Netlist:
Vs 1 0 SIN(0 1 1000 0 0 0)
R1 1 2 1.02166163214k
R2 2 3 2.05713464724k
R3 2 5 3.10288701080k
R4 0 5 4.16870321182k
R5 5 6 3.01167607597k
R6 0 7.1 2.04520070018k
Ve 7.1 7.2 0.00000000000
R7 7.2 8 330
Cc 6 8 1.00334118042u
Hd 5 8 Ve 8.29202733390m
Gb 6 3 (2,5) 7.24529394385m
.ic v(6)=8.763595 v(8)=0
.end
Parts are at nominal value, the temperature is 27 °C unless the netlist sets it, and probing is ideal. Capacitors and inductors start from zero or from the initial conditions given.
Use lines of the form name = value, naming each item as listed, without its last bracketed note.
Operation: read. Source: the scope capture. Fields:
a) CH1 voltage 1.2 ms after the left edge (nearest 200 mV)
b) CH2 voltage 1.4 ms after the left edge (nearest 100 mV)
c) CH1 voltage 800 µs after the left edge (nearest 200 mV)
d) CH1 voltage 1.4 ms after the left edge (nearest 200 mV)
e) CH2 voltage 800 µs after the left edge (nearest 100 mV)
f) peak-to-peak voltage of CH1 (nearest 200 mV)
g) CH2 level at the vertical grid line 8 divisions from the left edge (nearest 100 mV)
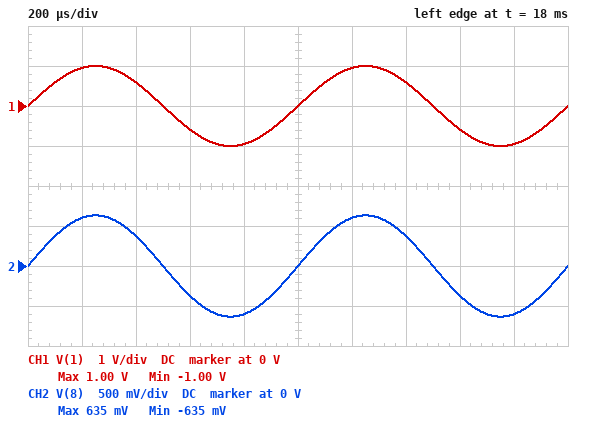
CH1 voltage 1.2 ms after the left edge = 1.0 V
CH2 voltage 1.4 ms after the left edge = 400 mV
CH1 voltage 800 µs after the left edge = -1.0 V
CH1 voltage 1.4 ms after the left edge = 600 mV
CH2 voltage 800 µs after the left edge = -600 mV
peak-to-peak voltage of CH1 = 2.0 V
CH2 level at the vertical grid line 8 divisions from the left edge = -400 mV
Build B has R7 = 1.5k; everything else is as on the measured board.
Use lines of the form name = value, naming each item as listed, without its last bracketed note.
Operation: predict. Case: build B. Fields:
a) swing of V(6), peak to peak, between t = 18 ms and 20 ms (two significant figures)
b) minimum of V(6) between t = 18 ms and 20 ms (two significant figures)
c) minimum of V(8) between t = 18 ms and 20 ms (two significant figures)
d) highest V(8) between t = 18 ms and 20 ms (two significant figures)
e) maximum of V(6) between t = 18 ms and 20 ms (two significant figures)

swing of V(6), peak to peak, between t = 18 ms and 20 ms = 1.4 V
minimum of V(6) between t = 18 ms and 20 ms = -680 mV
minimum of V(8) between t = 18 ms and 20 ms = -690 mV
highest V(8) between t = 18 ms and 20 ms = 690 mV
maximum of V(6) between t = 18 ms and 20 ms = 710 mV
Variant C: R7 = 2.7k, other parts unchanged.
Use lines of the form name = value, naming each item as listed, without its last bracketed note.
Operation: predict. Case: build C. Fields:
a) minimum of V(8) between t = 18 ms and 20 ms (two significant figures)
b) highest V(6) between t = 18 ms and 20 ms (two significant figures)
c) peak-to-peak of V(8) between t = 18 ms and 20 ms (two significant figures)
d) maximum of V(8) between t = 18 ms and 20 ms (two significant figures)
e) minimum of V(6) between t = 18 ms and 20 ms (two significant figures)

minimum of V(8) between t = 18 ms and 20 ms = -720 mV
highest V(6) between t = 18 ms and 20 ms = 740 mV
peak-to-peak of V(8) between t = 18 ms and 20 ms = 1.4 V
maximum of V(8) between t = 18 ms and 20 ms = 720 mV
minimum of V(6) between t = 18 ms and 20 ms = -710 mV
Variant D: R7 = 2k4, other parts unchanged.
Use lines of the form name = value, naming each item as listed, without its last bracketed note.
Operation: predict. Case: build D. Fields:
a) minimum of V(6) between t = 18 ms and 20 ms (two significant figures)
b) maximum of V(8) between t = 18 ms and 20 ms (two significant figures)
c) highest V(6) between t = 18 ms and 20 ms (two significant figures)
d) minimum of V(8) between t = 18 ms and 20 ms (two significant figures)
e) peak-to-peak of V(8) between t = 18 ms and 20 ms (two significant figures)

minimum of V(6) between t = 18 ms and 20 ms = -700 mV
maximum of V(8) between t = 18 ms and 20 ms = 710 mV
highest V(6) between t = 18 ms and 20 ms = 740 mV
minimum of V(8) between t = 18 ms and 20 ms = -710 mV
peak-to-peak of V(8) between t = 18 ms and 20 ms = 1.4 V
